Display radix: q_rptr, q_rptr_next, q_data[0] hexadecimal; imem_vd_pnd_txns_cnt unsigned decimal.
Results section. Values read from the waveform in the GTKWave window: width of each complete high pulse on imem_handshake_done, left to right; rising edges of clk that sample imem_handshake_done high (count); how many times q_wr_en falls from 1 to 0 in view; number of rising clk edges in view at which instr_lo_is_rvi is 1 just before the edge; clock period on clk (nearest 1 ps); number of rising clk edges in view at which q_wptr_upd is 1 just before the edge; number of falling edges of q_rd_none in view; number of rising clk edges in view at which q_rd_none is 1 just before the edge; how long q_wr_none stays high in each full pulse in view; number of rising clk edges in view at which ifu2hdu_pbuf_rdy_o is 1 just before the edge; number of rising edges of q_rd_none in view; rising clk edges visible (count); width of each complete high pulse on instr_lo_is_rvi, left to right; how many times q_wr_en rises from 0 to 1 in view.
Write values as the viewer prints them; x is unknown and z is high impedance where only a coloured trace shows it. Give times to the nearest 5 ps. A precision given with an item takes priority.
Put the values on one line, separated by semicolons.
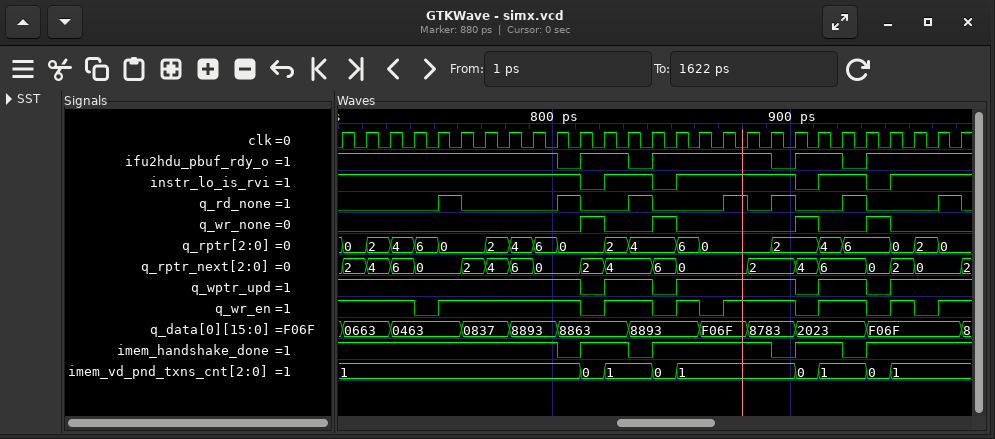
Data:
20 ps, 50 ps, 20 ps; 23; 7; 23; 10 ps; 23; 7; 7; 10 ps, 10 ps, 10 ps, 10 ps; 23; 7; 27; 20 ps, 50 ps, 20 ps; 7
